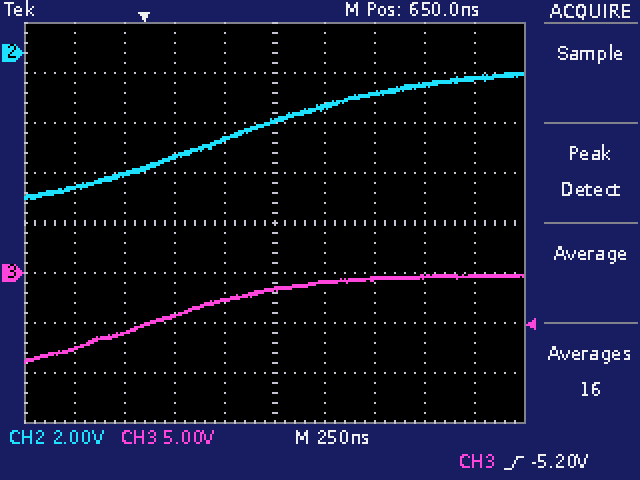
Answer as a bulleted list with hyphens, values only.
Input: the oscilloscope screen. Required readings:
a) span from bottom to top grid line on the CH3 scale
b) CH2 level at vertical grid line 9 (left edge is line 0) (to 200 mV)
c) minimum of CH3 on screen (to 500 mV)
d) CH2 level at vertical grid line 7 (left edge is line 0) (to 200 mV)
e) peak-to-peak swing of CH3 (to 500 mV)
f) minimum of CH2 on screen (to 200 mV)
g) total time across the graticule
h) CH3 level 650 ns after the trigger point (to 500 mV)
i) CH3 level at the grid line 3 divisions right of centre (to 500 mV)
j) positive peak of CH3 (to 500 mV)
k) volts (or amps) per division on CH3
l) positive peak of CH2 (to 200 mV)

- 40 V
- -1.0 V
- -9.0 V
- -1.6 V
- 9.0 V
- -5.8 V
- 2.5 µs
- -1.5 V
- -500 mV
- 0.0 V
- 5 V
- -800 mV
